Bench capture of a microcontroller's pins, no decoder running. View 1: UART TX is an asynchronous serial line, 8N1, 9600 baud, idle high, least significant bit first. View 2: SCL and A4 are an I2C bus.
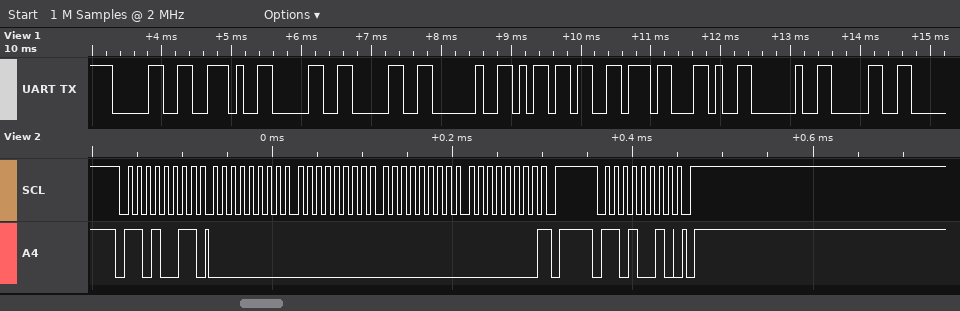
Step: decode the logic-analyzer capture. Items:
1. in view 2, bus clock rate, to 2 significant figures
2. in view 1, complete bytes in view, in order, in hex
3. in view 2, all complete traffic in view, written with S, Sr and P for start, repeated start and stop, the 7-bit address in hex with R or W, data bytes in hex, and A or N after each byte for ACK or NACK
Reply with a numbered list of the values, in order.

1. 100 kHz
2. 30 2E 30 30 20 6D 76 2C 20 30
3. S 69R A 00 A 00 A 00 A 00 N P S 69W A P
